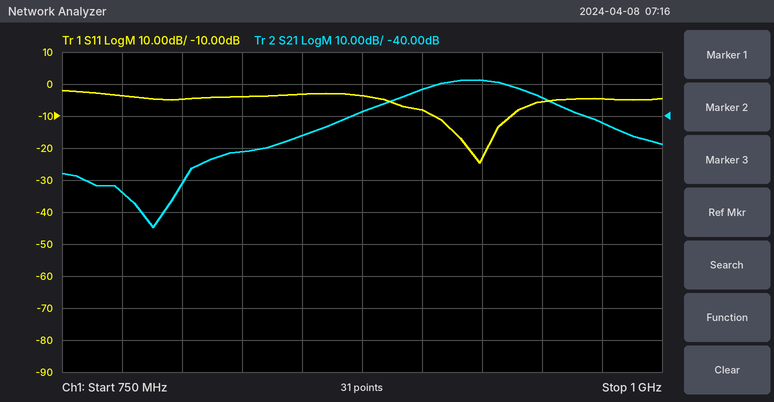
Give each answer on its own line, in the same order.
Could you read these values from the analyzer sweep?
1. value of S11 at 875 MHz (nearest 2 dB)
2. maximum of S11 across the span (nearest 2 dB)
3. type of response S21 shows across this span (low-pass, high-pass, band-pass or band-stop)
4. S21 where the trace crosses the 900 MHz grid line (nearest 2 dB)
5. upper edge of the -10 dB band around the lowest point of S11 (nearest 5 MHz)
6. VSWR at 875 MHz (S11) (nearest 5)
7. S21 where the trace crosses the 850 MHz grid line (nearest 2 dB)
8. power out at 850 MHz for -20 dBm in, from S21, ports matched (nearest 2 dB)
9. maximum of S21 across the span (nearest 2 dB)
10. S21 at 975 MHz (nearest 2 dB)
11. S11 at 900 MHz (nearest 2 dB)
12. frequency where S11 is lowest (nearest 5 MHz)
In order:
-4 dB
-2 dB
band-pass
-32 dB
935 MHz
5
-46 dB
-66 dBm
-28 dB
-42 dB
-8 dB
925 MHz
